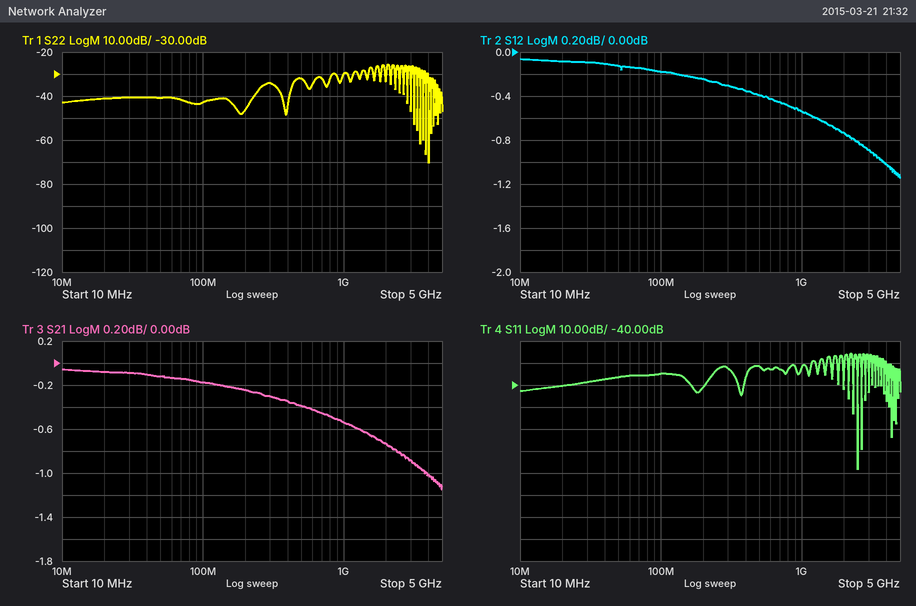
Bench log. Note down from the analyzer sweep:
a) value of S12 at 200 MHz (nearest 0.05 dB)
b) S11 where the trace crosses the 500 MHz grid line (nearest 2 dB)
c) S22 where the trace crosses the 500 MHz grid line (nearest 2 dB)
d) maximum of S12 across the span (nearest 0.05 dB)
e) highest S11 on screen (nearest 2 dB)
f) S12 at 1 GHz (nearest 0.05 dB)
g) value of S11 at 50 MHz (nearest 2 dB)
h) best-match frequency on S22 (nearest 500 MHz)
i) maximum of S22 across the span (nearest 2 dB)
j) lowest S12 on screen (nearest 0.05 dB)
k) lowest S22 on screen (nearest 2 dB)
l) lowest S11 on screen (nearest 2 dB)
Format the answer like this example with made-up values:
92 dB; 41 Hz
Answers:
-0.25 dB; -32 dB; -32 dB; -0.05 dB; -26 dB; -0.55 dB; -36 dB; 4.0 GHz; -26 dB; -1.15 dB; -70 dB; -78 dB
